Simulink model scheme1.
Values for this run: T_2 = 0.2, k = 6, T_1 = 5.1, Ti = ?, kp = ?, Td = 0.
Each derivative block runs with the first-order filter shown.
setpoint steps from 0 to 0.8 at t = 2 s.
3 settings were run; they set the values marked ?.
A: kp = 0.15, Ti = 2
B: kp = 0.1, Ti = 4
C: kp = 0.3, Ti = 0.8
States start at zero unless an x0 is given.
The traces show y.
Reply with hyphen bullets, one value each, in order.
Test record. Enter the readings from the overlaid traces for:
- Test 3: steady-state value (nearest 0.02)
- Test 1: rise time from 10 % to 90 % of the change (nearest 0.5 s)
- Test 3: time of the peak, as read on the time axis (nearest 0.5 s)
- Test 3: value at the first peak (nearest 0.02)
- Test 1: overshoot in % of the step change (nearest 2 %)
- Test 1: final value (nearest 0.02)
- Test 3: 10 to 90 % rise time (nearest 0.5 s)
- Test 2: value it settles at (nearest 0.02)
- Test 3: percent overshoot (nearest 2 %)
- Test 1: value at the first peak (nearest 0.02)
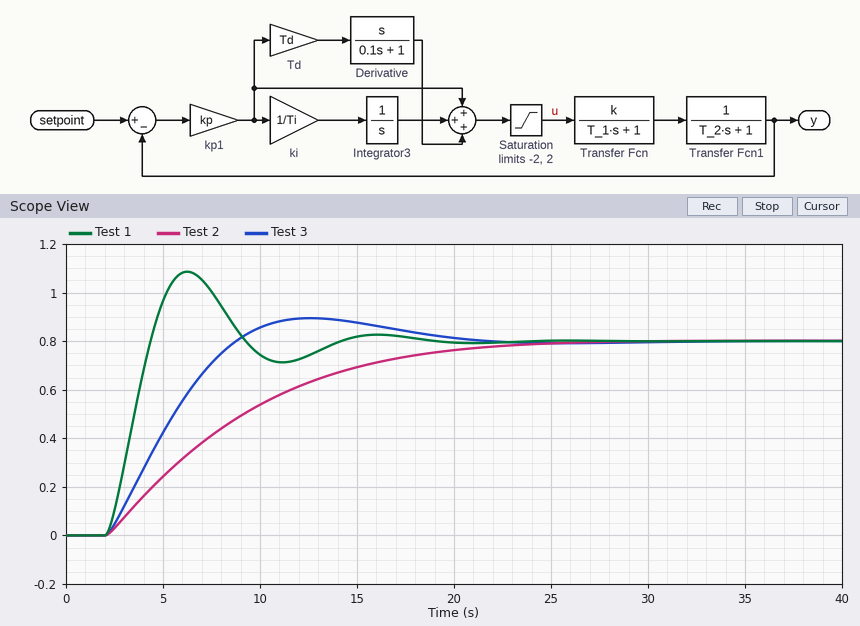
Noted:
- 0.80
- 1.5 s
- 12.5 s
- 0.90
- 36 %
- 0.80
- 5.0 s
- 0.80
- 12 %
- 1.08
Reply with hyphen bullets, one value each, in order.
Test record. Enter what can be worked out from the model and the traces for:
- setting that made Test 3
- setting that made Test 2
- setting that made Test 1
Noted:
- A
- B
- C
